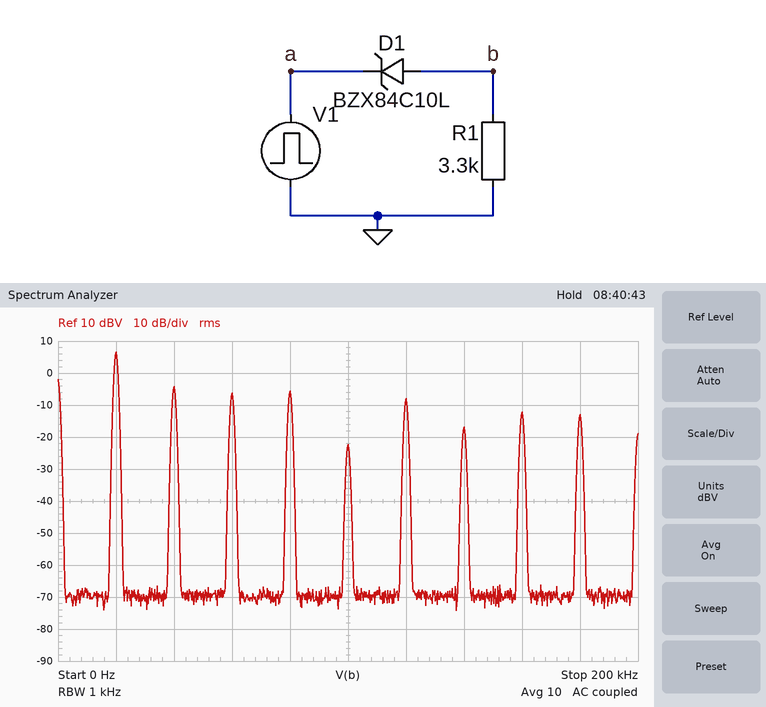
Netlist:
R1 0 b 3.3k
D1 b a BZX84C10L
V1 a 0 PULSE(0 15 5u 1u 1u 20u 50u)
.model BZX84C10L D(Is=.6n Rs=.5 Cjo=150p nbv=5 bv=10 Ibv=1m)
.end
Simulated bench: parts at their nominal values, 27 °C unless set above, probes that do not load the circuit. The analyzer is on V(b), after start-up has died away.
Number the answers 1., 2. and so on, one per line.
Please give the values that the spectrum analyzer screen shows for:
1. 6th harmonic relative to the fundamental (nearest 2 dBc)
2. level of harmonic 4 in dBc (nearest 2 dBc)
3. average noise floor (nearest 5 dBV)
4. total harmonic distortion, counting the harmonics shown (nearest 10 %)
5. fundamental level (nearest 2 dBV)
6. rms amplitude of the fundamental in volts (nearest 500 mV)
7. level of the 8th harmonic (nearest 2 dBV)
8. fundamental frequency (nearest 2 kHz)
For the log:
1. -14 dBc
2. -12 dBc
3. -70 dBV
4. 50 %
5. 6 dBV
6. 2.0 V
7. -12 dBV
8. 20 kHz
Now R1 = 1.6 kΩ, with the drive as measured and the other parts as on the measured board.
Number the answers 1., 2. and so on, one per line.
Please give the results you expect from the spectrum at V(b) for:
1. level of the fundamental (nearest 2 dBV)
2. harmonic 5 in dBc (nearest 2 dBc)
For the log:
1. 6 dBV
2. -32 dBc
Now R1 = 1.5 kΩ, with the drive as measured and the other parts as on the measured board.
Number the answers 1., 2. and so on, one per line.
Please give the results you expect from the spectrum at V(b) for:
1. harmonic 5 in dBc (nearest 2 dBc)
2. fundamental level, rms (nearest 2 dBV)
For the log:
1. -32 dBc
2. 6 dBV
